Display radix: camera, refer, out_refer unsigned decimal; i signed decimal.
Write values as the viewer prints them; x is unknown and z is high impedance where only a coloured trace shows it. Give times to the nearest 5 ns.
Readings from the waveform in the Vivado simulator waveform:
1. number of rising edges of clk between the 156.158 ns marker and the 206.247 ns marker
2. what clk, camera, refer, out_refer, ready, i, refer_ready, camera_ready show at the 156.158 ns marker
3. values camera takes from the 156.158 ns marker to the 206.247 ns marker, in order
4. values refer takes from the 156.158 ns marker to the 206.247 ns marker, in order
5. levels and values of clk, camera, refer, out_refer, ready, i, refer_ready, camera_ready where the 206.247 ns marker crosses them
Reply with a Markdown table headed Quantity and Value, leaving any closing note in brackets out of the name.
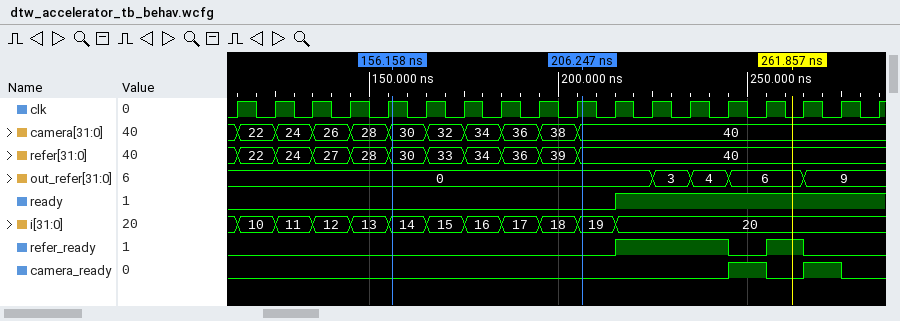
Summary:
| Quantity | Value |
|---|---|
| number of rising edges of clk between the 156.158 ns marker and the 206.247 ns marker | 5 |
| what clk, camera, refer, out_refer, ready, i, refer_ready, camera_ready show at the 156.158 ns marker | clk=1, camera=30, refer=30, out_refer=0, ready=0, i=14, refer_ready=0, camera_ready=0 |
| values camera takes from the 156.158 ns marker to the 206.247 ns marker, in order | 30, 32, 34, 36, 38, 40 |
| values refer takes from the 156.158 ns marker to the 206.247 ns marker, in order | 30, 33, 34, 36, 39, 40 |
| levels and values of clk, camera, refer, out_refer, ready, i, refer_ready, camera_ready where the 206.247 ns marker crosses them | clk=1, camera=40, refer=40, out_refer=0, ready=0, i=19, refer_ready=0, camera_ready=0 |
